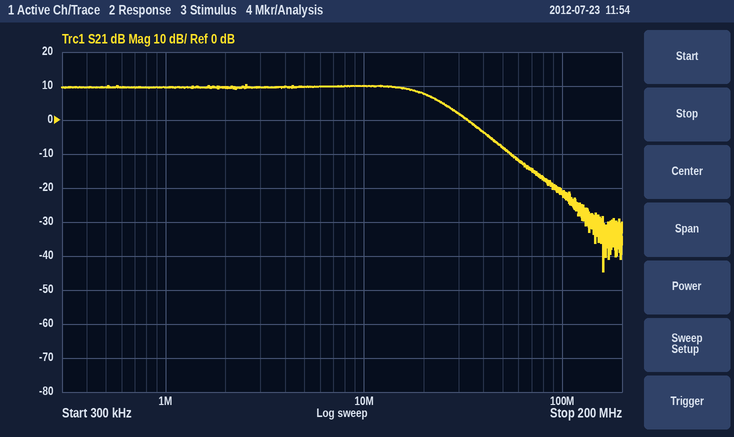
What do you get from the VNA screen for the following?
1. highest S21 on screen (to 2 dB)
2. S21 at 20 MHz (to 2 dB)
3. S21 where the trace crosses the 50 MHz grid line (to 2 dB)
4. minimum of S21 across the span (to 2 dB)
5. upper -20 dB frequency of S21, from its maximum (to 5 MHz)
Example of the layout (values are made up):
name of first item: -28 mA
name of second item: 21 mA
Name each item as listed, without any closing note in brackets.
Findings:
highest S21 on screen: 10 dB
S21 at 20 MHz: 8 dB
S21 where the trace crosses the 50 MHz grid line: -8 dB
minimum of S21 across the span: -44 dB
upper -20 dB frequency of S21, from its maximum: 55 MHz
